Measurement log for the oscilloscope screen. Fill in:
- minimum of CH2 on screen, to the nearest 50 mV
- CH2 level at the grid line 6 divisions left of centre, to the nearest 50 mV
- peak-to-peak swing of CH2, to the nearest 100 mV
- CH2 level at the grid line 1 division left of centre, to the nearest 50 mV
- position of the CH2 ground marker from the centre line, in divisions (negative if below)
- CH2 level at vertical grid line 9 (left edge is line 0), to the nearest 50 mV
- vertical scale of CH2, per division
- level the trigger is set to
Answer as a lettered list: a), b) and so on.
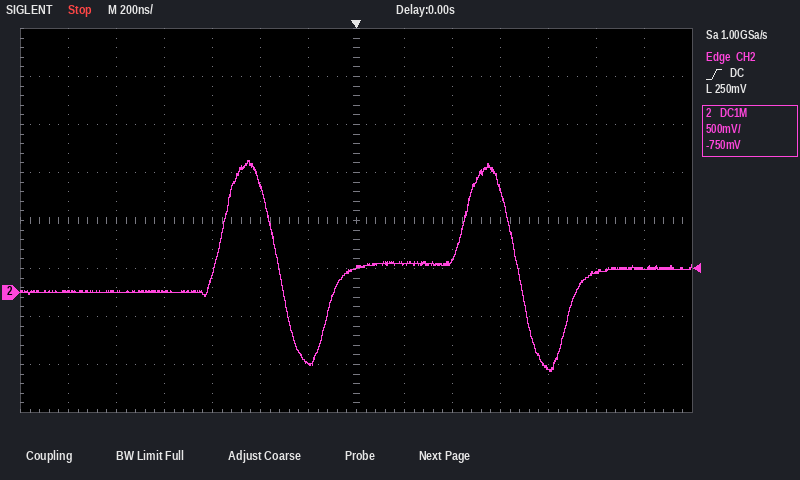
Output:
a) -800 mV
b) 0 mV
c) 2.20 V
d) -750 mV
e) -1.5 div
f) 350 mV
g) 500 mV
h) 250 mV
